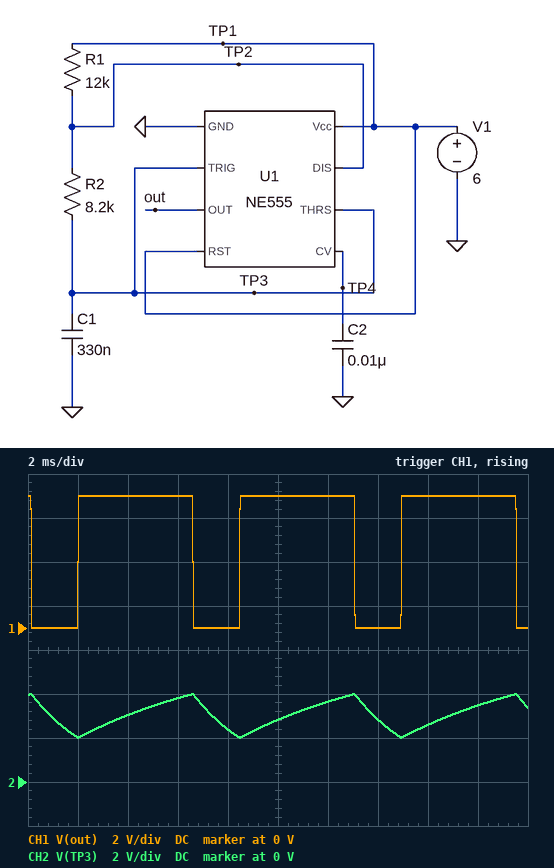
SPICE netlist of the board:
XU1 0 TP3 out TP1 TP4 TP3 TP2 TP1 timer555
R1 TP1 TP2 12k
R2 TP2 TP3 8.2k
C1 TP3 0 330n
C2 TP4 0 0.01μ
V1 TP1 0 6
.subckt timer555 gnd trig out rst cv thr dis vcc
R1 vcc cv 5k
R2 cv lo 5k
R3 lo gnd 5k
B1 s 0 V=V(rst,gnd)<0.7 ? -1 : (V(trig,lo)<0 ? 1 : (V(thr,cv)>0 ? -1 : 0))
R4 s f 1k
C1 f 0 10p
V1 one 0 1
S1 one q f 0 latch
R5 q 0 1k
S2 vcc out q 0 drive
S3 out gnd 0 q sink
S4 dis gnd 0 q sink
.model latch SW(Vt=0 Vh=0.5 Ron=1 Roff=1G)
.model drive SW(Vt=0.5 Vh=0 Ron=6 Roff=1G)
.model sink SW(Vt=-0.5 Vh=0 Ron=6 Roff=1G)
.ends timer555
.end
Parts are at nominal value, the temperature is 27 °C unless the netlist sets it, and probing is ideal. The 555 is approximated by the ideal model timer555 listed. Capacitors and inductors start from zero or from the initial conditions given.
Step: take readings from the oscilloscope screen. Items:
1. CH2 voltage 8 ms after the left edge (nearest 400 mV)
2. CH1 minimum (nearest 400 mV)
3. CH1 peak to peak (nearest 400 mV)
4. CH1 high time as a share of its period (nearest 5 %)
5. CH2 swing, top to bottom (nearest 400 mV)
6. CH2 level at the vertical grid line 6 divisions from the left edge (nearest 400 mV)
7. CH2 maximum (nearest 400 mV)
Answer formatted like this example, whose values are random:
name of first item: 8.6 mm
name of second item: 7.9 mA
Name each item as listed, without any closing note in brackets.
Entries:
CH2 voltage 8 ms after the left edge: 2.4 V
CH1 minimum: 0 V
CH1 peak to peak: 6.0 V
CH1 high time as a share of its period: 70 %
CH2 swing, top to bottom: 2.0 V
CH2 level at the vertical grid line 6 divisions from the left edge: 3.6 V
CH2 maximum: 4.0 V
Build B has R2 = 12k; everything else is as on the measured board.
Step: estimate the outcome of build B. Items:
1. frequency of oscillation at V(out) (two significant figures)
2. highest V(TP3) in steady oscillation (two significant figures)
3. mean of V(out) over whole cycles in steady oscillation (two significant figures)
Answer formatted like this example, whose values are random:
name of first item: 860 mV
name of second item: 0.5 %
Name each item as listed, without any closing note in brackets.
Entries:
frequency of oscillation at V(out): 120 Hz
highest V(TP3) in steady oscillation: 4.0 V
mean of V(out) over whole cycles in steady oscillation: 4.0 V
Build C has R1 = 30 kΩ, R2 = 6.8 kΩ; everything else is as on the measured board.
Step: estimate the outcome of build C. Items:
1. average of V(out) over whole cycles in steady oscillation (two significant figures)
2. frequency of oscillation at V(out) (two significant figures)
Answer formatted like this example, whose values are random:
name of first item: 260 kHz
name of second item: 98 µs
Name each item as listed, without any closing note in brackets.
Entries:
average of V(out) over whole cycles in steady oscillation: 5.1 V
frequency of oscillation at V(out): 100 Hz
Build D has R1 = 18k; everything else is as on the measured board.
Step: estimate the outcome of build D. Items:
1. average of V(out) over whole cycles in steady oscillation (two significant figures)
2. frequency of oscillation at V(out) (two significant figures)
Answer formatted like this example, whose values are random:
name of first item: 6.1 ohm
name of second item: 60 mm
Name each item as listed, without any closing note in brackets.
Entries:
average of V(out) over whole cycles in steady oscillation: 4.6 V
frequency of oscillation at V(out): 130 Hz
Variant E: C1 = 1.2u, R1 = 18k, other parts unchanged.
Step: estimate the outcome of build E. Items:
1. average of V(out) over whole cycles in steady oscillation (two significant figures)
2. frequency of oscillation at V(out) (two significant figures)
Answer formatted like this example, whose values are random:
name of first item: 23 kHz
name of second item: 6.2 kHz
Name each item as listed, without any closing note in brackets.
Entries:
average of V(out) over whole cycles in steady oscillation: 4.6 V
frequency of oscillation at V(out): 35 Hz
